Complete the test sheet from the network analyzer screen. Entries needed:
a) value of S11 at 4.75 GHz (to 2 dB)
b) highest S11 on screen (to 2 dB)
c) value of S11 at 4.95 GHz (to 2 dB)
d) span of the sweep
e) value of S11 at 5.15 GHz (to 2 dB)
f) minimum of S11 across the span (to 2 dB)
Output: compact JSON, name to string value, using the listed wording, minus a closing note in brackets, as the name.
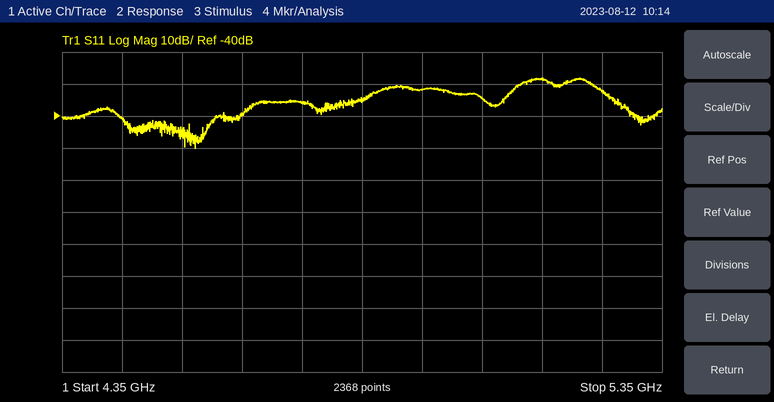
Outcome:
{"value of S11 at 4.75 GHz": "-36 dB", "highest S11 on screen": "-28 dB", "value of S11 at 4.95 GHz": "-32 dB", "span of the sweep": "1 GHz", "value of S11 at 5.15 GHz": "-28 dB", "minimum of S11 across the span": "-50 dB"}
